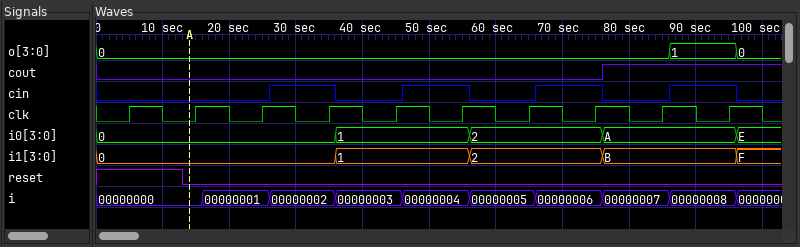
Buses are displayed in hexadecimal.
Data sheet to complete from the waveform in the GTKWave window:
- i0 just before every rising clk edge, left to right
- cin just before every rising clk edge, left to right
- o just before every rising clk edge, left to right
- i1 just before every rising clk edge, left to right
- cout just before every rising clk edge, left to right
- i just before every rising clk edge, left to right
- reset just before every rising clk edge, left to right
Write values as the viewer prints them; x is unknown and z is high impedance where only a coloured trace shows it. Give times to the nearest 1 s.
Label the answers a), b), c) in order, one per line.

a) 0, 0, 0, 0, 1, 1, 2, 2, A, A
b) 0 0 0 1 0 1 0 1 0 1
c) 0, 0, 0, 0, 0, 0, 0, 0, 0, 1
d) 0, 0, 0, 0, 1, 1, 2, 2, B, B
e) 0 0 0 0 0 0 0 0 1 1
f) 00000000, 00000000, 00000001, 00000002, 00000003, 00000004, 00000005, 00000006, 00000007, 00000008
g) 1 0 0 0 0 0 0 0 0 0
